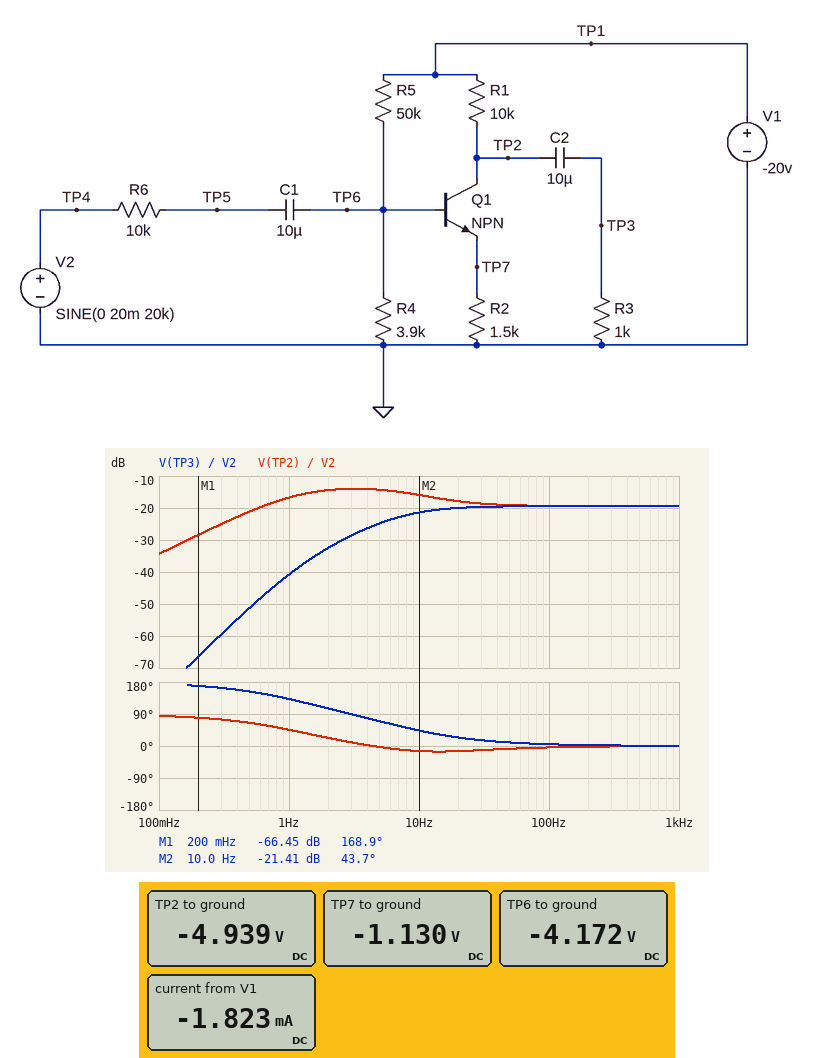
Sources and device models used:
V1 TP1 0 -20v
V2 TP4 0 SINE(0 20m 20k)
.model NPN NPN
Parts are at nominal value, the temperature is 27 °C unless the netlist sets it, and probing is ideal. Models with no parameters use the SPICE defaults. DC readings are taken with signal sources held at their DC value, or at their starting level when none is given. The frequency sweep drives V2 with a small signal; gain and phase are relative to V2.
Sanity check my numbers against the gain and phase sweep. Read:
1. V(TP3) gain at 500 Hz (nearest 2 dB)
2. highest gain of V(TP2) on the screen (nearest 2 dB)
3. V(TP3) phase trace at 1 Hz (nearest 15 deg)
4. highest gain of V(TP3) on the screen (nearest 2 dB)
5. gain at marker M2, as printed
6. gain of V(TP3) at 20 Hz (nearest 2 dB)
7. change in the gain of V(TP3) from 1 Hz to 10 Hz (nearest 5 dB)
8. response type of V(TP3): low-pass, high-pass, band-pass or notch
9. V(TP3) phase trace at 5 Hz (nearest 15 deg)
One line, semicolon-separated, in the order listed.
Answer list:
-20 dB; -14 dB; 135 deg; -20 dB; -21.41 dB; -20 dB; 20 dB; high-pass; 75 deg
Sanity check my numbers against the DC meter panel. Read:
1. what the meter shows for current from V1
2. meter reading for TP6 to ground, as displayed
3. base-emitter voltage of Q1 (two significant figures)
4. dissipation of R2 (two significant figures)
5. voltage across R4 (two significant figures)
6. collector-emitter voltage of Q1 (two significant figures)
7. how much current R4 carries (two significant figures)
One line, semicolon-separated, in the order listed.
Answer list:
-1.823 mA; -4.172 V; -3.0 V; 850 µW; 4.2 V; -3.8 V; 1.1 mA
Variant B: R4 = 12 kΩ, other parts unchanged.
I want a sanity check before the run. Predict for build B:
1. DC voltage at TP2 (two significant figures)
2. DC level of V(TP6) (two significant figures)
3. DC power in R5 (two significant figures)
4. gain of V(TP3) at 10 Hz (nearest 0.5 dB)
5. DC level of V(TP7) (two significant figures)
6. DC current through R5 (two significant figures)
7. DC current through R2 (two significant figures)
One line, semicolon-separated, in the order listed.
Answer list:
-9.6 V; -8.9 V; 2.5 mW; -19.0 dB; -780 mV; 220 µA; 520 µA
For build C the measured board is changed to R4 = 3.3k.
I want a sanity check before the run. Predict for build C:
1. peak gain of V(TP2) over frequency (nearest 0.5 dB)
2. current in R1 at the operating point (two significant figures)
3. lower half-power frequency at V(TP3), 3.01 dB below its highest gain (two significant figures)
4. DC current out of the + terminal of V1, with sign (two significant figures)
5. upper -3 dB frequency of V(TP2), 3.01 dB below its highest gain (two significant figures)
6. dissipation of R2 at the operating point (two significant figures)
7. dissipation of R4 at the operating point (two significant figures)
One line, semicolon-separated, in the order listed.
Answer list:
-15.0 dB; 1.6 mA; 8.1 Hz; -1.9 mA; 16 Hz; 910 µW; 4.0 mW
